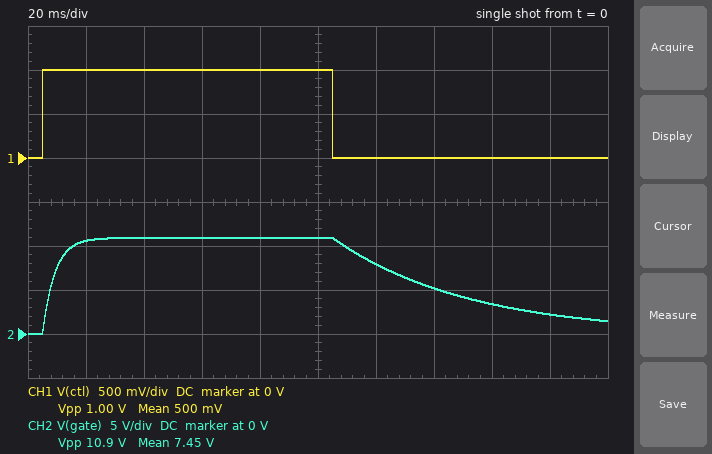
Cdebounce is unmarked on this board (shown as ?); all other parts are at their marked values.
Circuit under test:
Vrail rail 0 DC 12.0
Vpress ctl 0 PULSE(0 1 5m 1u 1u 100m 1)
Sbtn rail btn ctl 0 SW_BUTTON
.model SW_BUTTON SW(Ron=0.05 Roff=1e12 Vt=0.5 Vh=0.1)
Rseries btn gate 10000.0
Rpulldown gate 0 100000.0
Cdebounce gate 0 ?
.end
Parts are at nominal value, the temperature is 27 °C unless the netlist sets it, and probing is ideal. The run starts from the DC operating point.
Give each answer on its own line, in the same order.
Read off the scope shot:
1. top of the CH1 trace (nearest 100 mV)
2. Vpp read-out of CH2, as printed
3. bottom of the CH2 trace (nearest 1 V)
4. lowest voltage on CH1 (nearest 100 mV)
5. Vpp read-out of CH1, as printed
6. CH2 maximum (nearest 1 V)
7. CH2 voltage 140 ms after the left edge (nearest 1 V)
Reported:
1.0 V
10.9 V
0 V
0 V
1.00 V
11 V
5 V
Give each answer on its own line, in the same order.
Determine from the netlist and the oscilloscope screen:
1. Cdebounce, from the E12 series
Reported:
470 nF
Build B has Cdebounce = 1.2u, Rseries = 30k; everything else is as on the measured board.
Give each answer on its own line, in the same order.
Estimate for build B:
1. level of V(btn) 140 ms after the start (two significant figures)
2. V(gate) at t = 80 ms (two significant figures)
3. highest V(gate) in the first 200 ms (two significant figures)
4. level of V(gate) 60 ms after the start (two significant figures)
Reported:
6.7 V
8.6 V
9.0 V
8.0 V
